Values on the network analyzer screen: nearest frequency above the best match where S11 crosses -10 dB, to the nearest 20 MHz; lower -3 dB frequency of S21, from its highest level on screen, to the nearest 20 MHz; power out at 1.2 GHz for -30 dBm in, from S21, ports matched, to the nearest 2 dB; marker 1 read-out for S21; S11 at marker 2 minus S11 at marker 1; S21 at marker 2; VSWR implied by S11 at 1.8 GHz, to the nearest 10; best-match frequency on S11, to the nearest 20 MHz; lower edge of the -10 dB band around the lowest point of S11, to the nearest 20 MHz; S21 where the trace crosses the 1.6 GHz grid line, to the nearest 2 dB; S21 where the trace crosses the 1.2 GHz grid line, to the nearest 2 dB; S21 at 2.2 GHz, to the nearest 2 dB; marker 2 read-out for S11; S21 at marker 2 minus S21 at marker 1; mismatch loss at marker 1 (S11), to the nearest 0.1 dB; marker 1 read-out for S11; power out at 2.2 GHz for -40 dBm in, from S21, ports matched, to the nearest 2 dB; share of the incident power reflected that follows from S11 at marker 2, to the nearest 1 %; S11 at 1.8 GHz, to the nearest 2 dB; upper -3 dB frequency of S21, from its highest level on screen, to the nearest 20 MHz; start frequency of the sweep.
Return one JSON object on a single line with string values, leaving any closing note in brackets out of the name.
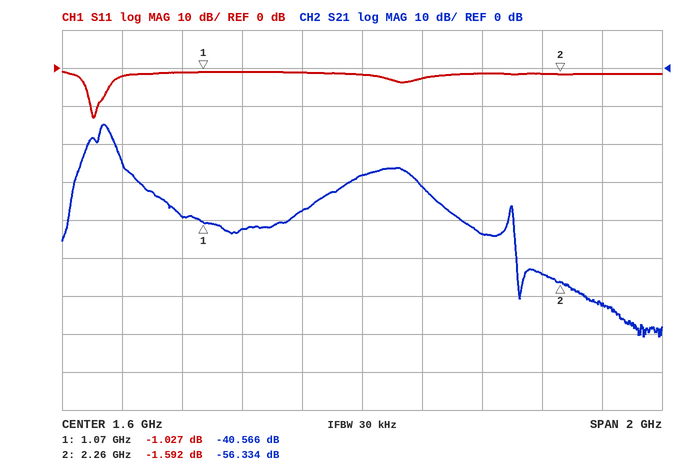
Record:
{"nearest frequency above the best match where S11 crosses -10 dB, to the nearest 20 MHz": "720 MHz", "lower -3 dB frequency of S21, from its highest level on screen, to the nearest 20 MHz": "720 MHz", "power out at 1.2 GHz for -30 dBm in, from S21, ports matched, to the nearest 2 dB": "-72 dBm", "marker 1 read-out for S21": "-40.566 dB", "S11 at marker 2 minus S11 at marker 1": "-0.565 dB", "S21 at marker 2": "-56.334 dB", "VSWR implied by S11 at 1.8 GHz, to the nearest 10": "10", "best-match frequency on S11, to the nearest 20 MHz": "700 MHz", "lower edge of the -10 dB band around the lowest point of S11, to the nearest 20 MHz": "700 MHz", "S21 where the trace crosses the 1.6 GHz grid line, to the nearest 2 dB": "-28 dB", "S21 where the trace crosses the 1.2 GHz grid line, to the nearest 2 dB": "-42 dB", "S21 at 2.2 GHz, to the nearest 2 dB": "-54 dB", "marker 2 read-out for S11": "-1.592 dB", "S21 at marker 2 minus S21 at marker 1": "-15.768 dB", "mismatch loss at marker 1 (S11), to the nearest 0.1 dB": "6.8 dB", "marker 1 read-out for S11": "-1.027 dB", "power out at 2.2 GHz for -40 dBm in, from S21, ports matched, to the nearest 2 dB": "-94 dBm", "share of the incident power reflected that follows from S11 at marker 2, to the nearest 1 %": "69 %", "S11 at 1.8 GHz, to the nearest 2 dB": "-2 dB", "upper -3 dB frequency of S21, from its highest level on screen, to the nearest 20 MHz": "760 MHz", "start frequency of the sweep": "600 MHz"}
